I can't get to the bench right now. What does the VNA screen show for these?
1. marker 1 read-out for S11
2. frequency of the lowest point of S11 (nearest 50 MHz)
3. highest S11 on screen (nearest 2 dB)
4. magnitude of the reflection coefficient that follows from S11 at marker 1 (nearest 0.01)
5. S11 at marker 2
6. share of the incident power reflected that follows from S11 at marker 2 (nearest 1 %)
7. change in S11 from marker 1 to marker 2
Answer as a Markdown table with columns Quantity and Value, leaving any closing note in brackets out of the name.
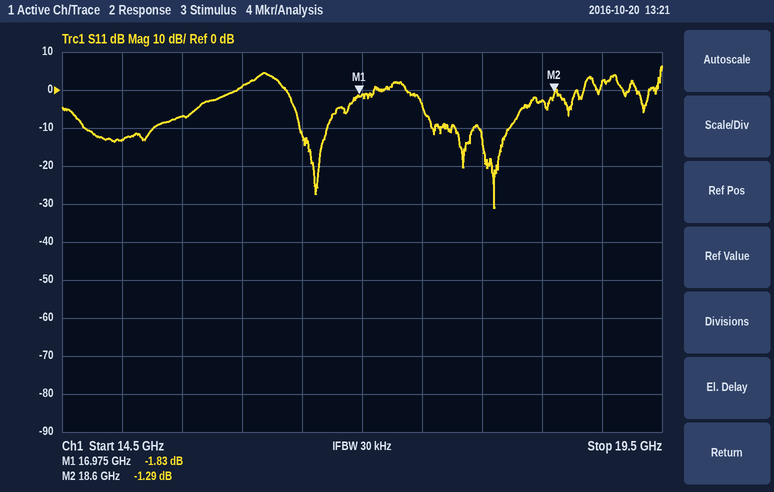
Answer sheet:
| Quantity | Value |
|---|---|
| marker 1 read-out for S11 | -1.83 dB |
| frequency of the lowest point of S11 | 18.10 GHz |
| highest S11 on screen | 6 dB |
| magnitude of the reflection coefficient that follows from S11 at marker 1 | 0.81 |
| S11 at marker 2 | -1.29 dB |
| share of the incident power reflected that follows from S11 at marker 2 | 74 % |
| change in S11 from marker 1 to marker 2 | 0.54 dB |
